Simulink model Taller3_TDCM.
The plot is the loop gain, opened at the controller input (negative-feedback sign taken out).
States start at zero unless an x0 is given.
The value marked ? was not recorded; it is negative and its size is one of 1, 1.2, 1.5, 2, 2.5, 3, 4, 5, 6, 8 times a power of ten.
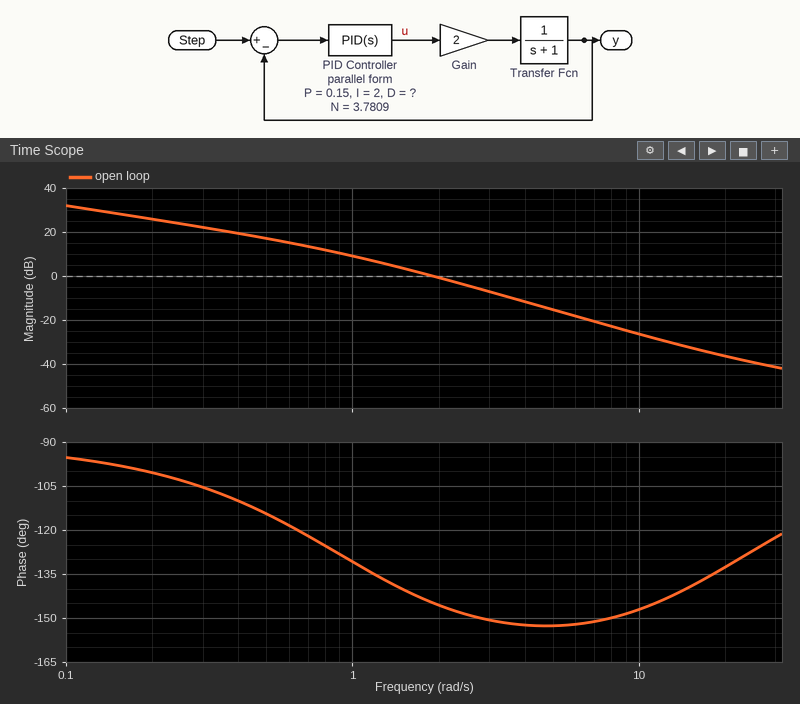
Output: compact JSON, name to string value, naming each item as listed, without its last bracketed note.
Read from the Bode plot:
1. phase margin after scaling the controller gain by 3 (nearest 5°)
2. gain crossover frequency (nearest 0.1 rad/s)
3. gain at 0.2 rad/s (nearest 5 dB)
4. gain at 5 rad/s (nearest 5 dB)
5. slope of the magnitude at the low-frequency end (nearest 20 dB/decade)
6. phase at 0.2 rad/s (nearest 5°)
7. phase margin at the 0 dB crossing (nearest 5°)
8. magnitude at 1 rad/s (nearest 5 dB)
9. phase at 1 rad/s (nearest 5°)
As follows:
{"phase margin after scaling the controller gain by 3": "30°", "gain crossover frequency": "1.9 rad/s", "gain at 0.2 rad/s": "25 dB", "gain at 5 rad/s": "-15 dB", "slope of the magnitude at the low-frequency end": "-20 dB/decade", "phase at 0.2 rad/s": "-100°", "phase margin at the 0 dB crossing": "35°", "magnitude at 1 rad/s": "10 dB", "phase at 1 rad/s": "-130°"}
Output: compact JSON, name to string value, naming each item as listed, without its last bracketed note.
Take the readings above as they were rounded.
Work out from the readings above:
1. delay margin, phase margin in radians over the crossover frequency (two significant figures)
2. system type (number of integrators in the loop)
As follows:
{"delay margin, phase margin in radians over the crossover frequency": "0.32 s", "system type": "1"}
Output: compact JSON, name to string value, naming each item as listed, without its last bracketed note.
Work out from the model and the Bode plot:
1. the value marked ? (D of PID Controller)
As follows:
{"the value marked ?": "-0.012"}
